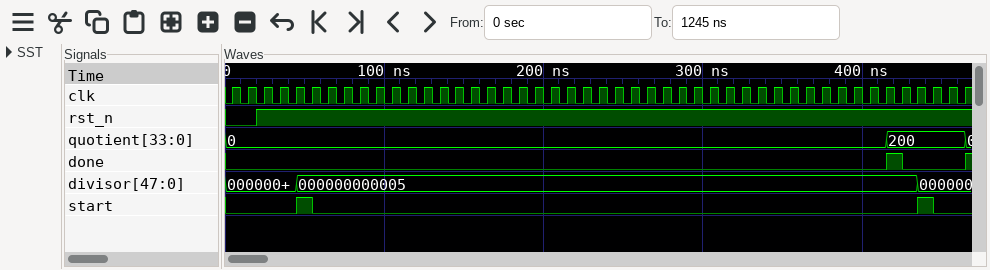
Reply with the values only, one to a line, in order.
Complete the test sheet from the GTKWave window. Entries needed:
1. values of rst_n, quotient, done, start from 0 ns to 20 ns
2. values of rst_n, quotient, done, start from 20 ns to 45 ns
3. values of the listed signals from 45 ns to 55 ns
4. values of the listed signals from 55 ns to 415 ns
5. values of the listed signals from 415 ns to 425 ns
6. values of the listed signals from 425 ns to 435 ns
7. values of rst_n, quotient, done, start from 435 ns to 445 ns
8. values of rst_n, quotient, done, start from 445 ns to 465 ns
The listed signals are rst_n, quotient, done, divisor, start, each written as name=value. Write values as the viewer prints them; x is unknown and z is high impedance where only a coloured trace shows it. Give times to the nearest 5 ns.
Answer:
rst_n=0, quotient=0, done=0, start=0
rst_n=1, quotient=0, done=0, start=0
rst_n=1, quotient=0, done=0, divisor=000000000005, start=1
rst_n=1, quotient=0, done=0, divisor=000000000005, start=0
rst_n=1, quotient=200, done=1, divisor=000000000005, start=0
rst_n=1, quotient=200, done=0, divisor=000000000005, start=0
rst_n=1, quotient=200, done=0, start=1
rst_n=1, quotient=200, done=0, start=0
